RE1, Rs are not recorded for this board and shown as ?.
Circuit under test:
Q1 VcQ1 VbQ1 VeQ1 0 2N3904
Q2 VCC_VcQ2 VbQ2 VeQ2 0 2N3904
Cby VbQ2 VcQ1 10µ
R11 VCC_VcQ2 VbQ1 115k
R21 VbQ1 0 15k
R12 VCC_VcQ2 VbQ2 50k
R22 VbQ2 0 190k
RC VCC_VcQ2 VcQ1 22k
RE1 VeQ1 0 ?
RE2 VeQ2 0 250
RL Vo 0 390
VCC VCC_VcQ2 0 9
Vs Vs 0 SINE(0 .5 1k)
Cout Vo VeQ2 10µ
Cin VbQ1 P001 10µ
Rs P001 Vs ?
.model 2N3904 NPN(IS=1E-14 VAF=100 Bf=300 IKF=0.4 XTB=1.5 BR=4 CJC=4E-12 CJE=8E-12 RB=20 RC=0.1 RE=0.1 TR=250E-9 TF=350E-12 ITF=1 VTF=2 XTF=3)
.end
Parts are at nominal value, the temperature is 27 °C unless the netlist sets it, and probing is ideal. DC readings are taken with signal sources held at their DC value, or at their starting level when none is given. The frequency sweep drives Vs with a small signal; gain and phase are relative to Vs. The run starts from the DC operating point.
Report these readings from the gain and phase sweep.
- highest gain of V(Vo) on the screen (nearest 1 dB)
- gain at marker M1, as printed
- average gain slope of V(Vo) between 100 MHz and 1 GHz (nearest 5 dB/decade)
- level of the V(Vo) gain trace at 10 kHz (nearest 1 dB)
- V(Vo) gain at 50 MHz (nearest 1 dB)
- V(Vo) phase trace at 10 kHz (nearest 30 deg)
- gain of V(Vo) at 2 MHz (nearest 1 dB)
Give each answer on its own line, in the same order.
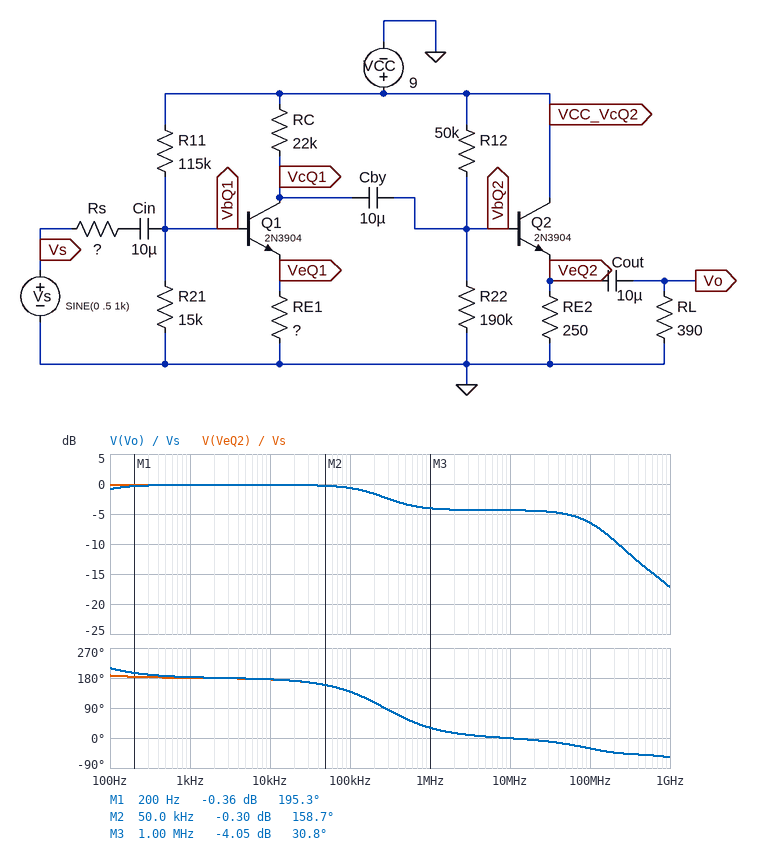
0 dB
-0.36 dB
-10 dB/decade
0 dB
-5 dB
180 deg
-4 dB
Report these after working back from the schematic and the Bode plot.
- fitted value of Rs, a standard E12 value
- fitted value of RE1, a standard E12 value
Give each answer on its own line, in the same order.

330 Ω
560 Ω
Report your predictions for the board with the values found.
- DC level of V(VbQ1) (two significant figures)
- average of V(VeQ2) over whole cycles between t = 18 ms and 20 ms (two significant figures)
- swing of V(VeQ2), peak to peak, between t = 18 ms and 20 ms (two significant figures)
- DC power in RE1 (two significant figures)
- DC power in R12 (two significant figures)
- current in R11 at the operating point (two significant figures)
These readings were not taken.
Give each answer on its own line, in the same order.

860 mV
6.3 V
4.4 V
94 µW
330 µW
71 µA
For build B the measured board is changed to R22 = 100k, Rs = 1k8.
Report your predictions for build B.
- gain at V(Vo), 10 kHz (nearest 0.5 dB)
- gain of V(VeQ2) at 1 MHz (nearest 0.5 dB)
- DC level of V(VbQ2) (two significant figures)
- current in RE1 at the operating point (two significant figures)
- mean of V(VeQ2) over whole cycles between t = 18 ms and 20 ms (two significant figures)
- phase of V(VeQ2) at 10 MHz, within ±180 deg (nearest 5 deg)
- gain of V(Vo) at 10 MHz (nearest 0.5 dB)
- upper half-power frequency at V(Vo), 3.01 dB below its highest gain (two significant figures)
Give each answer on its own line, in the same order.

-7.0 dB
-12.5 dB
4.4 V
410 µA
5.3 V
-5 deg
-13.0 dB
270 kHz
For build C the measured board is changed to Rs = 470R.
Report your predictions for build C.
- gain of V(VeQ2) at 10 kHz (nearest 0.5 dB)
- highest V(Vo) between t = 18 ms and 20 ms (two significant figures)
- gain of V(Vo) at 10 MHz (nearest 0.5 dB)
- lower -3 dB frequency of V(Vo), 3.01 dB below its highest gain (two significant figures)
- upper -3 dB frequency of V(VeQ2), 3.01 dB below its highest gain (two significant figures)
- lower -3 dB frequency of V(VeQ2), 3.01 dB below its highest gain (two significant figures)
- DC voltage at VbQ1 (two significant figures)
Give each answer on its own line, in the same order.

-1.0 dB
2.3 V
-5.5 dB
43 Hz
390 kHz
12 Hz
860 mV
